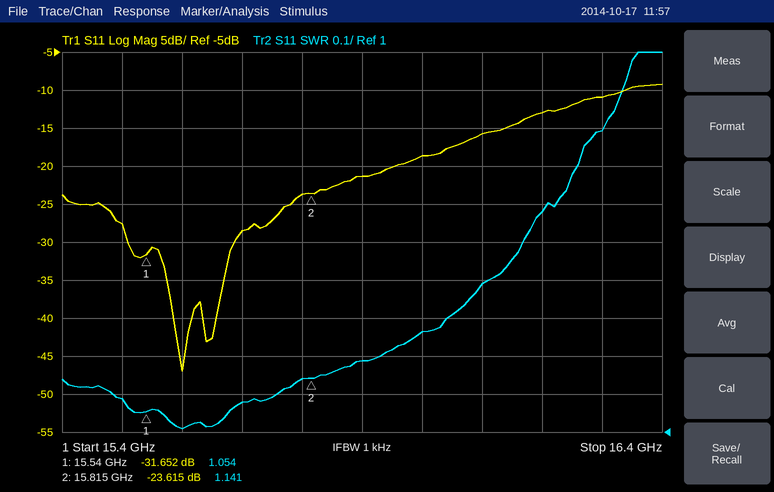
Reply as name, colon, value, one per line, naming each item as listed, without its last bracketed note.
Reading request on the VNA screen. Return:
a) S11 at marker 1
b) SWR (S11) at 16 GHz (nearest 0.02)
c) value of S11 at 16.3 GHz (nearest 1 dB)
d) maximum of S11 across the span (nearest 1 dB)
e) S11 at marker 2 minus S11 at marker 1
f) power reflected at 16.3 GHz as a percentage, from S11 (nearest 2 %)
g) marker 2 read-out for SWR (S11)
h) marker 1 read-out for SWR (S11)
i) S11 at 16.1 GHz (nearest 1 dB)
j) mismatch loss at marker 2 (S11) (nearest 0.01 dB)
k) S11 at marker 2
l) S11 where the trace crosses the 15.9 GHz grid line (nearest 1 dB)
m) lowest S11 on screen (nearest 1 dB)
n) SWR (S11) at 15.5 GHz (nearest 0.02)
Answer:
S11 at marker 1: -31.652 dB
SWR (S11) at 16 GHz: 1.26
value of S11 at 16.3 GHz: -11 dB
maximum of S11 across the span: -9 dB
S11 at marker 2 minus S11 at marker 1: 8.037 dB
power reflected at 16.3 GHz as a percentage, from S11: 8 %
marker 2 read-out for SWR: 1.141
marker 1 read-out for SWR: 1.054
S11 at 16.1 GHz: -16 dB
mismatch loss at marker 2 (S11): 0.02 dB
S11 at marker 2: -23.615 dB
S11 where the trace crosses the 15.9 GHz grid line: -21 dB
lowest S11 on screen: -47 dB
SWR (S11) at 15.5 GHz: 1.08
